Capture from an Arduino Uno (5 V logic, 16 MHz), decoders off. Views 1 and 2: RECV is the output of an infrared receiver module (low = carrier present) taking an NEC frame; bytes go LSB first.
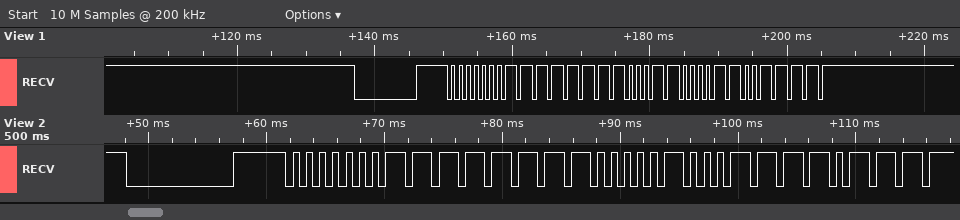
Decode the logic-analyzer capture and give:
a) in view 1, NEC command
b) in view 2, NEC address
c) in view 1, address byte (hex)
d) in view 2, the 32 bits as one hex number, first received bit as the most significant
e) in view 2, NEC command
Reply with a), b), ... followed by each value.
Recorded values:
a) 0x0C
b) 0x80
c) 0x80
d) 0x01FE08F7
e) 0x10
